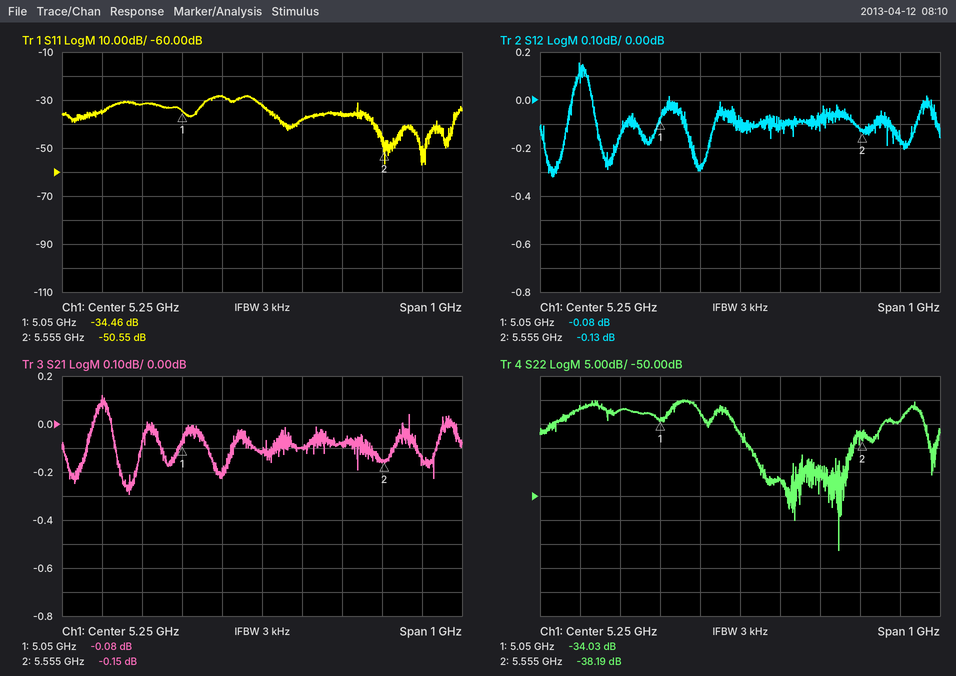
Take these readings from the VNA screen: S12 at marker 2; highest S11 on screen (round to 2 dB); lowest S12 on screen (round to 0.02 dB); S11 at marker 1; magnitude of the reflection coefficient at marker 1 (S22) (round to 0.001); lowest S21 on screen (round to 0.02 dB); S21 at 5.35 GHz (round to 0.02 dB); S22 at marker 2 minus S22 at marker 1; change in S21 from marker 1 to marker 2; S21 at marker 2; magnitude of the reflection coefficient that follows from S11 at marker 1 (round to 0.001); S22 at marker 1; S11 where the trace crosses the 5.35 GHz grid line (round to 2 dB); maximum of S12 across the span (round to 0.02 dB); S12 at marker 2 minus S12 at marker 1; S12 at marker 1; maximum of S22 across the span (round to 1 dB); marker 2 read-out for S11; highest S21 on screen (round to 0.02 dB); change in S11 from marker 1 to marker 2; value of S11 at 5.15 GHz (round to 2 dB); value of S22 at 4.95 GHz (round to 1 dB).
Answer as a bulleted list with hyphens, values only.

- -0.13 dB
- -28 dB
- -0.32 dB
- -34.46 dB
- 0.020
- -0.30 dB
- -0.10 dB
- -4.16 dB
- -0.07 dB
- -0.15 dB
- 0.019
- -34.03 dB
- -38 dB
- 0.16 dB
- -0.05 dB
- -0.08 dB
- -30 dB
- -50.55 dB
- 0.12 dB
- -16.09 dB
- -28 dB
- -32 dB
